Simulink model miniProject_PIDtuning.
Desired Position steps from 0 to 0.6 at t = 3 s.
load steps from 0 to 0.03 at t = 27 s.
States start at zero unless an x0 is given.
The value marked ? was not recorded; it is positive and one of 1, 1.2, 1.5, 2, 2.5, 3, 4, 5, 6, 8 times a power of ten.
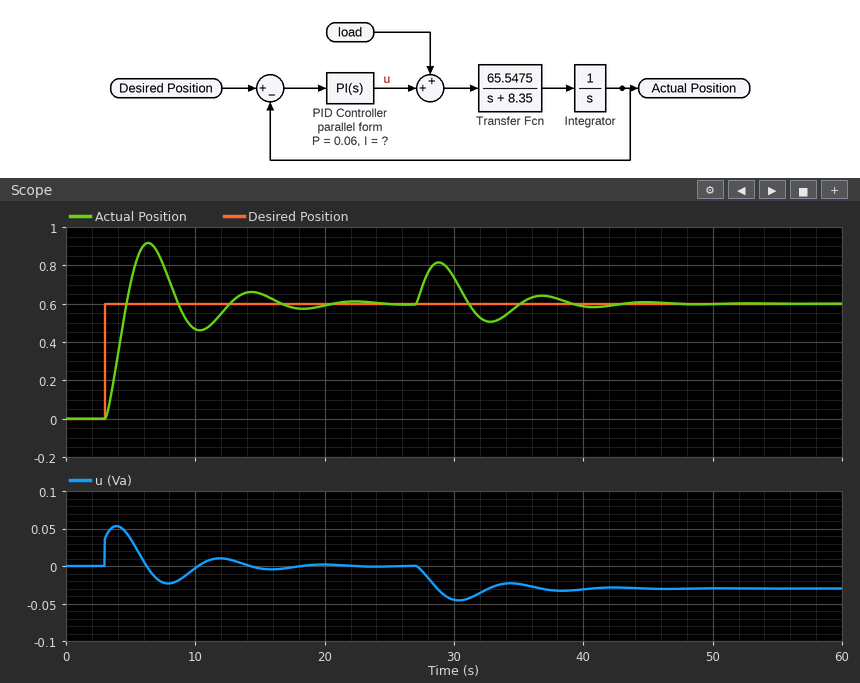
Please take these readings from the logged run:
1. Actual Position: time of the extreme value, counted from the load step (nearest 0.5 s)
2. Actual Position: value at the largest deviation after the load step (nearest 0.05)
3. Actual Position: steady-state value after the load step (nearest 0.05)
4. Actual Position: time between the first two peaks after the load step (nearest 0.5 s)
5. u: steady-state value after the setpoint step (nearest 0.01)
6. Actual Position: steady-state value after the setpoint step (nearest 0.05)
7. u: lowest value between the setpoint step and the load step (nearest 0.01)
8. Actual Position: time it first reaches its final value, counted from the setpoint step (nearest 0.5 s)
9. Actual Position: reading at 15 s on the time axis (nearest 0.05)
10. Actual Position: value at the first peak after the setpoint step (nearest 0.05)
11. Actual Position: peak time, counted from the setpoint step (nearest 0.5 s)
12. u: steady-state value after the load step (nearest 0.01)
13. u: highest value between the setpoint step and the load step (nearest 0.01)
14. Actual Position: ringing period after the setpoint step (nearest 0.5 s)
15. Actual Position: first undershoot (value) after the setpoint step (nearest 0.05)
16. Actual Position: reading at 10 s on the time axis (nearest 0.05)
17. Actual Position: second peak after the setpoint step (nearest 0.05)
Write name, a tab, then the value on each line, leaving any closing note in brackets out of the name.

Actual Position: time of the extreme value, counted from the load step	2.0 s
Actual Position: value at the largest deviation after the load step	0.80
Actual Position: steady-state value after the load step	0.60
Actual Position: time between the first two peaks after the load step	8.0 s
u: steady-state value after the setpoint step	0.00
Actual Position: steady-state value after the setpoint step	0.60
u: lowest value between the setpoint step and the load step	-0.02
Actual Position: time it first reaches its final value, counted from the setpoint step	1.5 s
Actual Position: reading at 15 s on the time axis	0.65
Actual Position: value at the first peak after the setpoint step	0.90
Actual Position: peak time, counted from the setpoint step	3.5 s
u: steady-state value after the load step	-0.03
u: highest value between the setpoint step and the load step	0.05
Actual Position: ringing period after the setpoint step	8.0 s
Actual Position: first undershoot (value) after the setpoint step	0.45
Actual Position: reading at 10 s on the time axis	0.45
Actual Position: second peak after the setpoint step	0.65
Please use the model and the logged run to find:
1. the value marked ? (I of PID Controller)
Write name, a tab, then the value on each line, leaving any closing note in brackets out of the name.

the value marked ?	0.08
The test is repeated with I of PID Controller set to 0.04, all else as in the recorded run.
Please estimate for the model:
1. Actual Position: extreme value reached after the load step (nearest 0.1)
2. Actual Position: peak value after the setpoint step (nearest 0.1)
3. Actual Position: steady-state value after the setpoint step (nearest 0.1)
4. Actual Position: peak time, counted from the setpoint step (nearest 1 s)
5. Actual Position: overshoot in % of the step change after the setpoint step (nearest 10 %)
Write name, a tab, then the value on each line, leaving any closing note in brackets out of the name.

Actual Position: extreme value reached after the load step	0.9
Actual Position: peak value after the setpoint step	0.8
Actual Position: steady-state value after the setpoint step	0.6
Actual Position: peak time, counted from the setpoint step	4 s
Actual Position: overshoot in % of the step change after the setpoint step	40 %
